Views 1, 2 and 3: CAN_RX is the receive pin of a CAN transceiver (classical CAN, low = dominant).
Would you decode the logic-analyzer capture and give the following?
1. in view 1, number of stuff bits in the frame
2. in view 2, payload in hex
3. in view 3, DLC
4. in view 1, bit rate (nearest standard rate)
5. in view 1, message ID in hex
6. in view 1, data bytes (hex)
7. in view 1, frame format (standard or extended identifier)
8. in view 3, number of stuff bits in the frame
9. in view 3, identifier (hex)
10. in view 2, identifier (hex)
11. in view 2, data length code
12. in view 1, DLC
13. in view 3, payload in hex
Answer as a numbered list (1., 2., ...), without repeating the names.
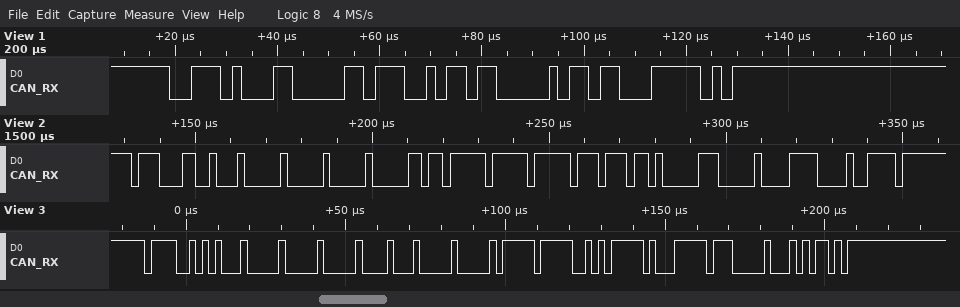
1. 3
2. 00 00 5B FF FF 76 83 00
3. 8
4. 500 kbit/s
5. 0x3A3
6. E5 B0
7. standard
8. 10
9. 0x795
10. 0x719
11. 8
12. 2
13. 00 00 88 00 FF D5 F8 FF
